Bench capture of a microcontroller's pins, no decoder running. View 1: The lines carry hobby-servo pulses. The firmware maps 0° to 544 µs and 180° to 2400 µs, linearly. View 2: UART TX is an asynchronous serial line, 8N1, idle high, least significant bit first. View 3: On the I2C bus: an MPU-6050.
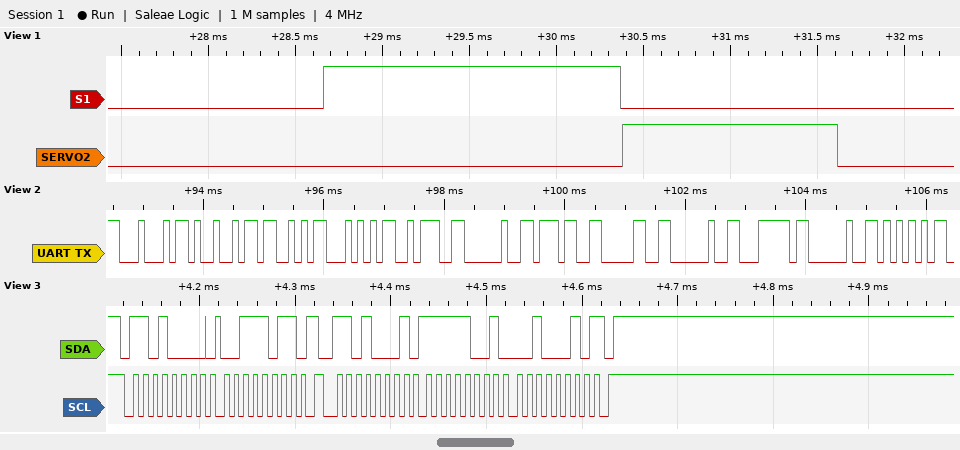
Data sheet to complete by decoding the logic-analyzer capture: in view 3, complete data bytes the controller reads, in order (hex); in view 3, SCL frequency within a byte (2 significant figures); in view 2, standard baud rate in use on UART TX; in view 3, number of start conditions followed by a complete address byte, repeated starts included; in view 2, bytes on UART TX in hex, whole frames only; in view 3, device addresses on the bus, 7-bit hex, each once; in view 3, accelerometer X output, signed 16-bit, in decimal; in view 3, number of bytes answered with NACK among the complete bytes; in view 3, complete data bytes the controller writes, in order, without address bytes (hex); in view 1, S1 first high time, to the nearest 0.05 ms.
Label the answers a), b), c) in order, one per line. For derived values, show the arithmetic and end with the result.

a) F9 22
b) 100 kHz
c) 9600 baud
d) 2
e) 44 49 53 54 3A 20 37 30 20 7C 20 55
f) 0x68
g) 0xF922 = -1758
h) 1
i) 3B
j) 1.70 ms
